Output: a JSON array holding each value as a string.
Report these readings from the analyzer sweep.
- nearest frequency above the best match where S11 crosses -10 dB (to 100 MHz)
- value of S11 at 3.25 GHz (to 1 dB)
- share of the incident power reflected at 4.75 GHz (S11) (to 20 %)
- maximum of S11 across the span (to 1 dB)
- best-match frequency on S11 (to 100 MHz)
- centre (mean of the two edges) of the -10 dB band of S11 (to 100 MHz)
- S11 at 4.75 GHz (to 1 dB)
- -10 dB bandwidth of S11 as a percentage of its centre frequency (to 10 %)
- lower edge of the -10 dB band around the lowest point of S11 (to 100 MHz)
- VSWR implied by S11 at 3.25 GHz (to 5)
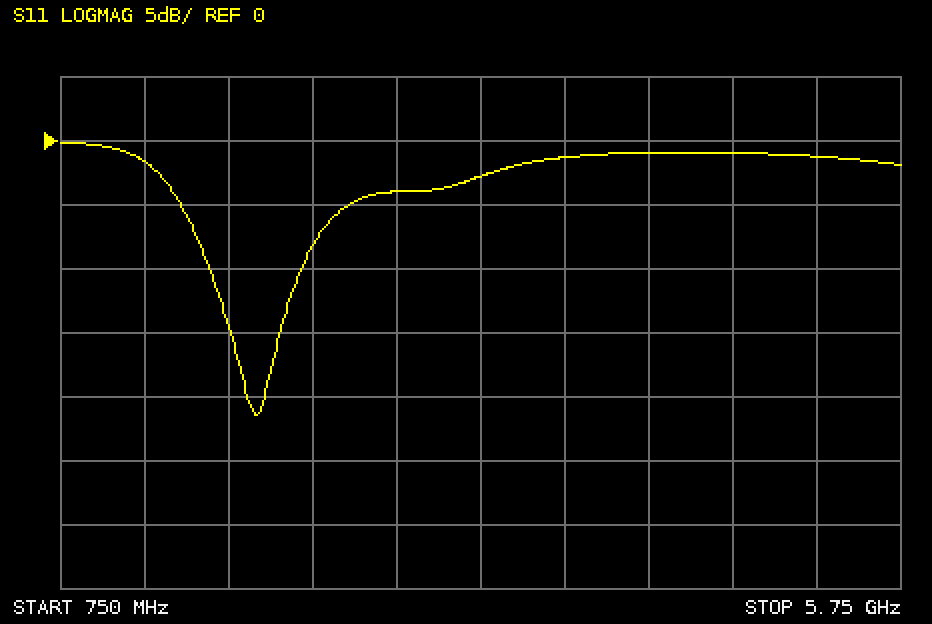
["2.2 GHz", "-3 dB", "80 %", "0 dB", "1.9 GHz", "1.9 GHz", "-1 dB", "30 %", "1.6 GHz", "5"]
